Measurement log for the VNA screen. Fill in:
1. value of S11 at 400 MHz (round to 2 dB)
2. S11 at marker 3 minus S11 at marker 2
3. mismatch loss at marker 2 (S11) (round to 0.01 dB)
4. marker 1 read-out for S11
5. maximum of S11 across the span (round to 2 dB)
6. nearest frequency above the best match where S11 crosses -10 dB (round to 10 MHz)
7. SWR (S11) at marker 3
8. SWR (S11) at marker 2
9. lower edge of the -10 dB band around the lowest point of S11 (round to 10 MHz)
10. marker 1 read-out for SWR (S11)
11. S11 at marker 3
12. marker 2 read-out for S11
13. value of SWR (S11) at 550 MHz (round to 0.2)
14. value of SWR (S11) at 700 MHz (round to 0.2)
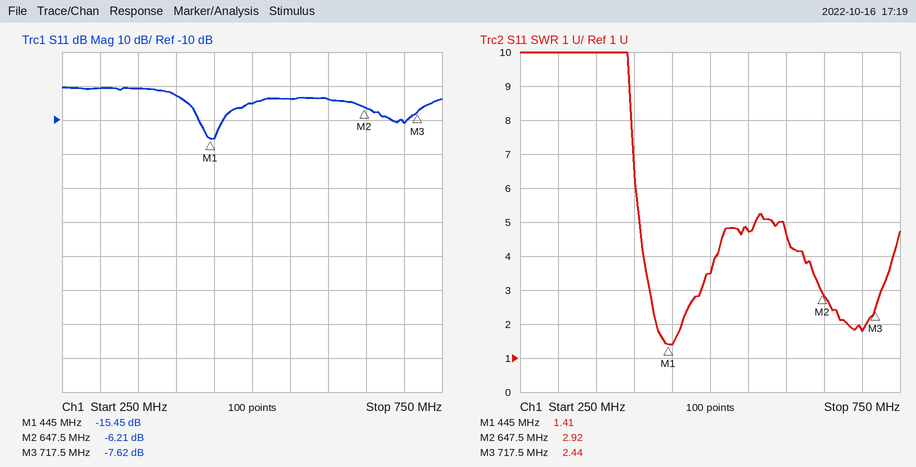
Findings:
-2 dB
-1.41 dB
1.19 dB
-15.45 dB
0 dB
460 MHz
2.44
2.92
430 MHz
1.41
-7.62 dB
-6.21 dB
4.8
1.8
